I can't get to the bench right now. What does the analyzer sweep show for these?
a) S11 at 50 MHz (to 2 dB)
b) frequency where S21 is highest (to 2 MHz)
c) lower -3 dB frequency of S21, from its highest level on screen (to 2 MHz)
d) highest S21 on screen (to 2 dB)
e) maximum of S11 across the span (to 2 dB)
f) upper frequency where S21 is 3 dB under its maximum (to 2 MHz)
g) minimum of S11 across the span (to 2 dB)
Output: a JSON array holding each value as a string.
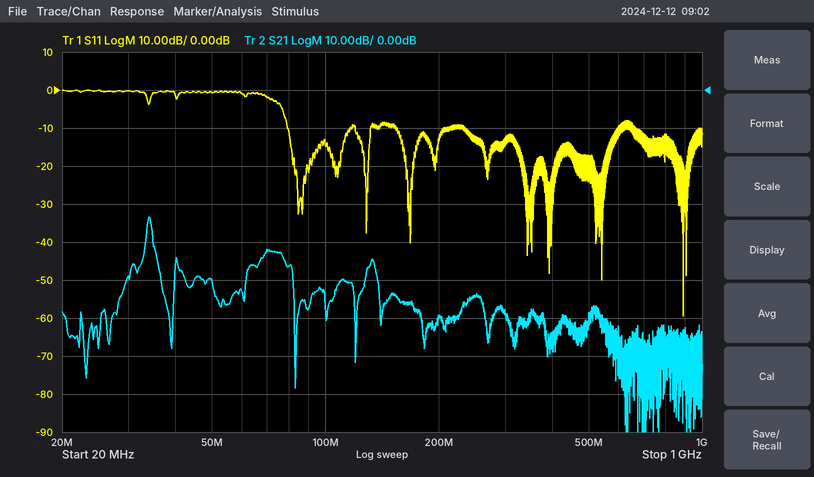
["0 dB", "34 MHz", "34 MHz", "-34 dB", "0 dB", "34 MHz", "-60 dB"]
